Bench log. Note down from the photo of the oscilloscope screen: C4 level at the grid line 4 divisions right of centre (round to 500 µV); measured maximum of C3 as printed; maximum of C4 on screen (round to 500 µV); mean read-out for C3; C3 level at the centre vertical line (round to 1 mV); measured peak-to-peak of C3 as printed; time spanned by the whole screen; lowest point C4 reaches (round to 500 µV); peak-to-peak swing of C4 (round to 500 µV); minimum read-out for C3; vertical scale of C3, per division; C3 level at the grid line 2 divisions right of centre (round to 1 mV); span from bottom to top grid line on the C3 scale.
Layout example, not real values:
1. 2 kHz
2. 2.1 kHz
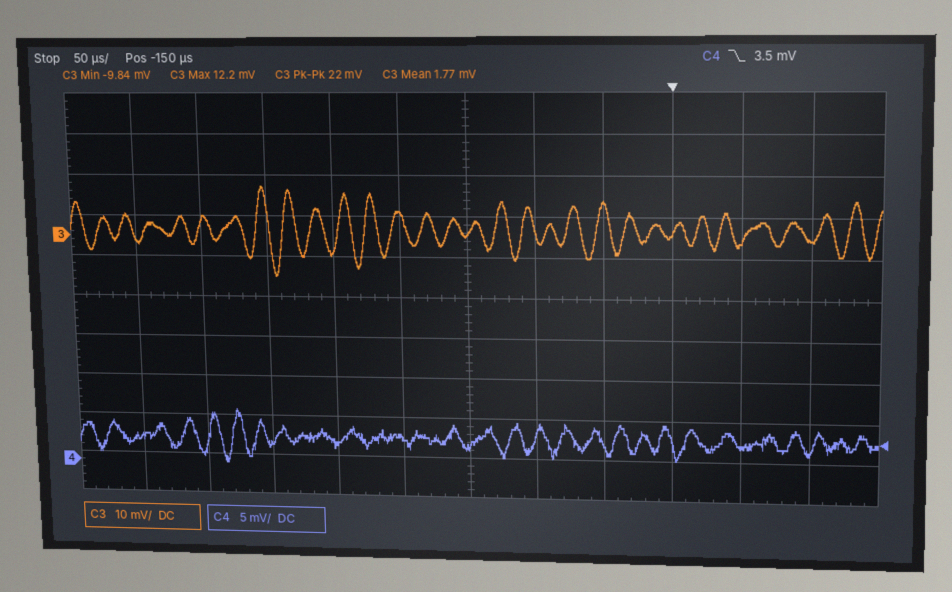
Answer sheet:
1. 3.0 mV
2. 12.2 mV
3. 6.5 mV
4. 1.77 mV
5. 1 mV
6. 22 mV
7. 600 µs
8. 0.0 mV
9. 6.5 mV
10. -9.84 mV
11. 10 mV
12. 8 mV
13. 100 mV
